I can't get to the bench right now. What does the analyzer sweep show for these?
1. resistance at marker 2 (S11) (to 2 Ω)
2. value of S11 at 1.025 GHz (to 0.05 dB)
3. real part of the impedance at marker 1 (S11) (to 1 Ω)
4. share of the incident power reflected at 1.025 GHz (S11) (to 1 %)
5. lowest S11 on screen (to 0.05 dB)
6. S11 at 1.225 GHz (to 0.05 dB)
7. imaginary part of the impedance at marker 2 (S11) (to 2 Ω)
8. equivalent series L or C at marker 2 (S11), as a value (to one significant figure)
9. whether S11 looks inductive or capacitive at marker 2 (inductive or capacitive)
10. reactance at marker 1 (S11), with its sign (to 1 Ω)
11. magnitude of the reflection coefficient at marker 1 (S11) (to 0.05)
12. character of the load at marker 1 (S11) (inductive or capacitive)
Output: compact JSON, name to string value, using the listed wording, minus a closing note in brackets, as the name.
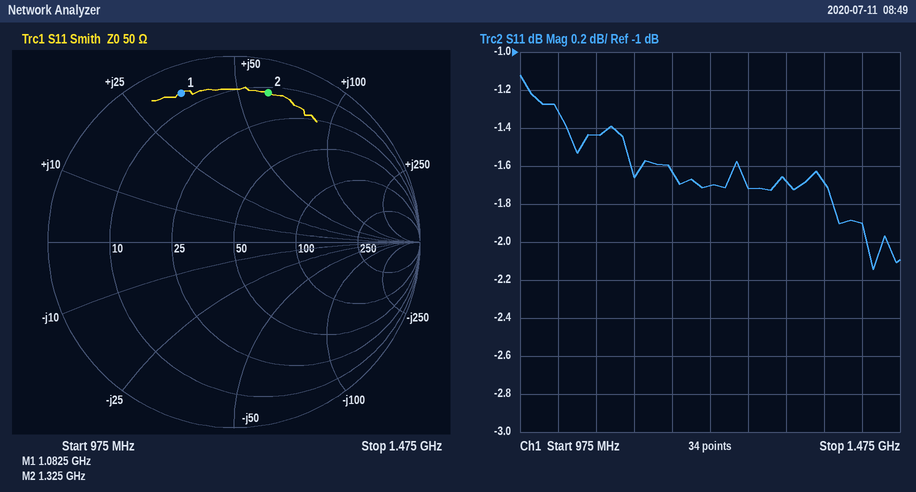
{"resistance at marker 2 (S11)": "12 Ω", "value of S11 at 1.025 GHz": "-1.30 dB", "real part of the impedance at marker 1 (S11)": "6 Ω", "share of the incident power reflected at 1.025 GHz (S11)": "74 %", "lowest S11 on screen": "-2.15 dB", "S11 at 1.225 GHz": "-1.70 dB", "imaginary part of the impedance at marker 2 (S11)": "+62 Ω", "equivalent series L or C at marker 2 (S11), as a value": "7 nH", "whether S11 looks inductive or capacitive at marker 2": "inductive", "reactance at marker 1 (S11), with its sign": "+35 Ω", "magnitude of the reflection coefficient at marker 1 (S11)": "0.85", "character of the load at marker 1 (S11)": "inductive"}
